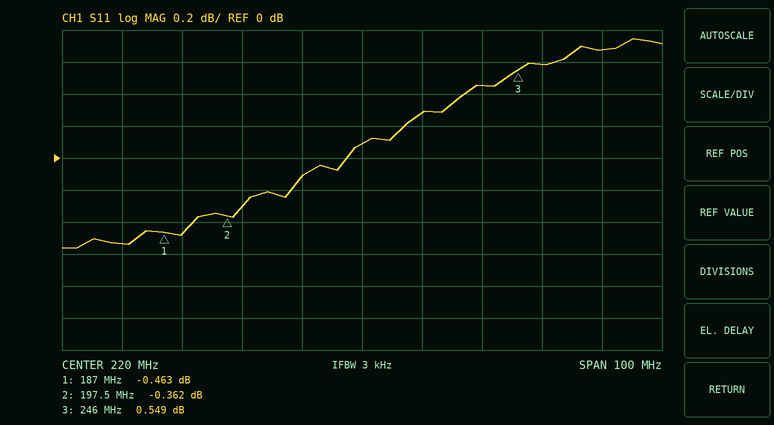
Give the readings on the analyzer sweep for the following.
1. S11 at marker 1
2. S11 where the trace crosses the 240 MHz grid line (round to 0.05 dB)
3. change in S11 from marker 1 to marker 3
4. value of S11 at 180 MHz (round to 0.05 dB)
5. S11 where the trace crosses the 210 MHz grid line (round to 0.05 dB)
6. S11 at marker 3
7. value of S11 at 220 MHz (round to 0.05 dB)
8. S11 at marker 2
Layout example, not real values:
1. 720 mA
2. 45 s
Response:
1. -0.463 dB
2. 0.45 dB
3. 1.012 dB
4. -0.55 dB
5. -0.10 dB
6. 0.549 dB
7. 0.10 dB
8. -0.362 dB
